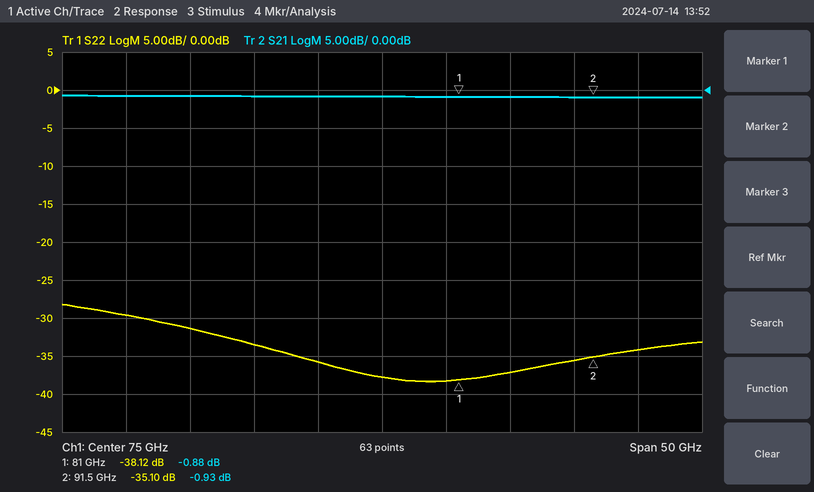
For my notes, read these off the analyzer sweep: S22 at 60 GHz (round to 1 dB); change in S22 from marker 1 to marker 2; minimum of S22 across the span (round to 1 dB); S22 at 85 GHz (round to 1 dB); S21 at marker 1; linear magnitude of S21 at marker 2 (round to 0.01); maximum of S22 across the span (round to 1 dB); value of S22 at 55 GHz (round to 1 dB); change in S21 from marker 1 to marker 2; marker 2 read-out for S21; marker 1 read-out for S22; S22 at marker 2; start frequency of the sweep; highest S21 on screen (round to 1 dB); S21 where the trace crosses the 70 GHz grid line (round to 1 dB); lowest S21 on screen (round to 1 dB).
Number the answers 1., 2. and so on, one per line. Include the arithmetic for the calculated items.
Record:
1. -31 dB
2. -35.1 − (-38.12) = 3.02 dB
3. -38 dB
4. -37 dB
5. -0.88 dB
6. 10^(-0.93/20) ≈ 0.90
7. -28 dB
8. -30 dB
9. -0.93 − (-0.88) = -0.05 dB
10. -0.93 dB
11. -38.12 dB
12. -35.10 dB
13. 50 GHz
14. -1 dB
15. -1 dB
16. -1 dB
